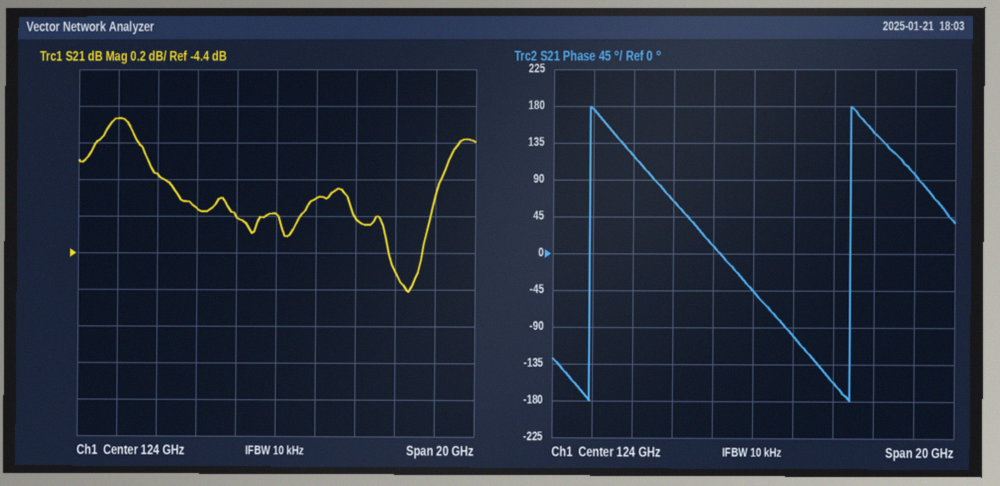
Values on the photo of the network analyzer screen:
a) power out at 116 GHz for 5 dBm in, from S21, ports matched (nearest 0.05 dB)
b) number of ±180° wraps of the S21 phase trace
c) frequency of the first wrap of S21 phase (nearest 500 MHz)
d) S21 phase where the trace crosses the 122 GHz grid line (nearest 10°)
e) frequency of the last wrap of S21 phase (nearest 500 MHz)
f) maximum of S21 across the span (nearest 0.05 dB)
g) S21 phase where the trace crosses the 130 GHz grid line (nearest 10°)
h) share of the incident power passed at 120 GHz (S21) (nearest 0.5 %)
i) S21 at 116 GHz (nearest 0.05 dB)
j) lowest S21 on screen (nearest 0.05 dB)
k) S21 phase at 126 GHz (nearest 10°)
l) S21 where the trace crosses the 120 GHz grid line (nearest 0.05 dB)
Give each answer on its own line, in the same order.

1.35 dBm
2
116.0 GHz
10°
129.0 GHz
-3.65 dB
150°
38.5 %
-3.65 dB
-4.60 dB
-100°
-4.15 dB
